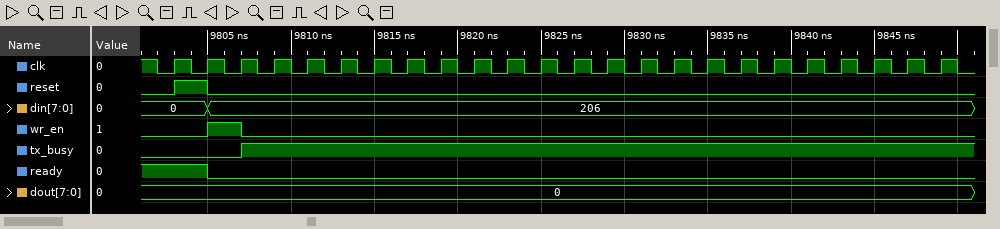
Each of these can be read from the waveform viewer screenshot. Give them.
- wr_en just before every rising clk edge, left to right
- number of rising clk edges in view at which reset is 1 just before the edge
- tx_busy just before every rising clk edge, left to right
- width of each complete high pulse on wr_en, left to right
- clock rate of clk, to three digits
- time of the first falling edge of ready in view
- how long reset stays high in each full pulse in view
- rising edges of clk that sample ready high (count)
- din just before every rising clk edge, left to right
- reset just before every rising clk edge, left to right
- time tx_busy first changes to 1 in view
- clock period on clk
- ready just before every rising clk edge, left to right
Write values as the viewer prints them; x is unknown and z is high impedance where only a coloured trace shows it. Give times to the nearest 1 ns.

0 0 1 0 0 0 0 0 0 0 0 0 0 0 0 0 0 0 0 0 0 0 0 0
1
0 0 0 1 1 1 1 1 1 1 1 1 1 1 1 1 1 1 1 1 1 1 1 1
2 ns
500 MHz
9805 ns
2 ns
2
0, 0, 206, 206, 206, 206, 206, 206, 206, 206, 206, 206, 206, 206, 206, 206, 206, 206, 206, 206, 206, 206, 206, 206
0 1 0 0 0 0 0 0 0 0 0 0 0 0 0 0 0 0 0 0 0 0 0 0
9807 ns
2 ns
1 1 0 0 0 0 0 0 0 0 0 0 0 0 0 0 0 0 0 0 0 0 0 0
